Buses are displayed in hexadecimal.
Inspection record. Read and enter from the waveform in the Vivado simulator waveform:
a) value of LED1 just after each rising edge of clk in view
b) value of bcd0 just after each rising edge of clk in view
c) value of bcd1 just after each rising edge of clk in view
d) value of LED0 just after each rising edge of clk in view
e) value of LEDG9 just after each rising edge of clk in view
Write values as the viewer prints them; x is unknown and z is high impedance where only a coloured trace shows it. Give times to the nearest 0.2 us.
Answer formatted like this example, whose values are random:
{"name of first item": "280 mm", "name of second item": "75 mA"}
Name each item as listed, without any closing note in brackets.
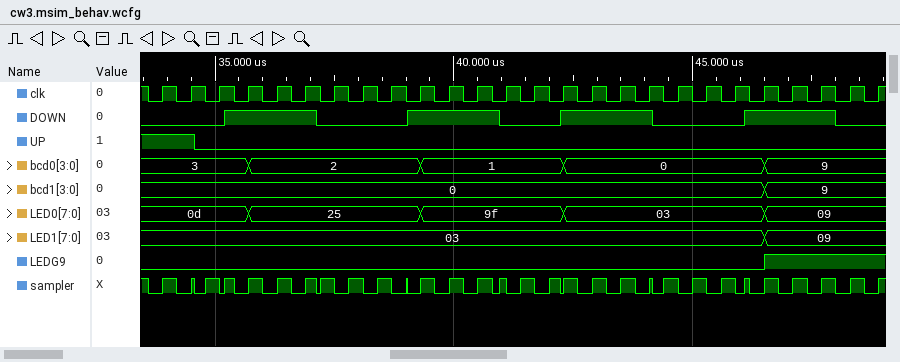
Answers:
{"value of LED1 just after each rising edge of clk in view": "03, 03, 03, 03, 03, 03, 03, 03, 03, 03, 03, 03, 03, 03, 03, 03, 03, 03, 03, 03, 03, 09, 09, 09, 09, 09", "value of bcd0 just after each rising edge of clk in view": "3, 3, 3, 2, 2, 2, 2, 2, 2, 1, 1, 1, 1, 1, 0, 0, 0, 0, 0, 0, 0, 9, 9, 9, 9, 9", "value of bcd1 just after each rising edge of clk in view": "0, 0, 0, 0, 0, 0, 0, 0, 0, 0, 0, 0, 0, 0, 0, 0, 0, 0, 0, 0, 0, 9, 9, 9, 9, 9", "value of LED0 just after each rising edge of clk in view": "0d, 0d, 0d, 25, 25, 25, 25, 25, 25, 9f, 9f, 9f, 9f, 9f, 03, 03, 03, 03, 03, 03, 03, 09, 09, 09, 09, 09", "value of LEDG9 just after each rising edge of clk in view": "0 0 0 0 0 0 0 0 0 0 0 0 0 0 0 0 0 0 0 0 0 1 1 1 1 1"}
